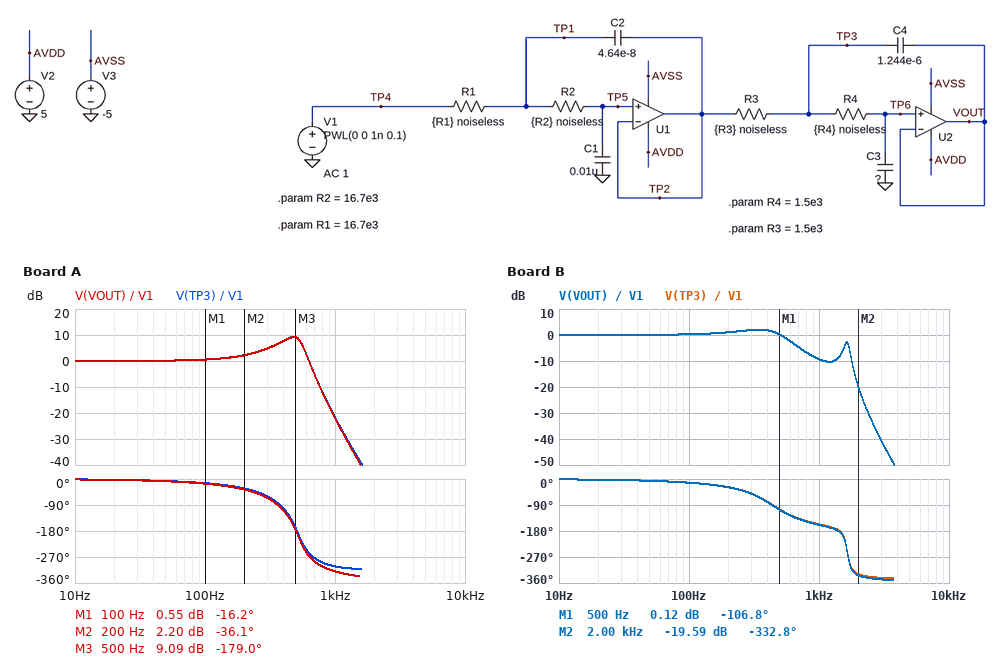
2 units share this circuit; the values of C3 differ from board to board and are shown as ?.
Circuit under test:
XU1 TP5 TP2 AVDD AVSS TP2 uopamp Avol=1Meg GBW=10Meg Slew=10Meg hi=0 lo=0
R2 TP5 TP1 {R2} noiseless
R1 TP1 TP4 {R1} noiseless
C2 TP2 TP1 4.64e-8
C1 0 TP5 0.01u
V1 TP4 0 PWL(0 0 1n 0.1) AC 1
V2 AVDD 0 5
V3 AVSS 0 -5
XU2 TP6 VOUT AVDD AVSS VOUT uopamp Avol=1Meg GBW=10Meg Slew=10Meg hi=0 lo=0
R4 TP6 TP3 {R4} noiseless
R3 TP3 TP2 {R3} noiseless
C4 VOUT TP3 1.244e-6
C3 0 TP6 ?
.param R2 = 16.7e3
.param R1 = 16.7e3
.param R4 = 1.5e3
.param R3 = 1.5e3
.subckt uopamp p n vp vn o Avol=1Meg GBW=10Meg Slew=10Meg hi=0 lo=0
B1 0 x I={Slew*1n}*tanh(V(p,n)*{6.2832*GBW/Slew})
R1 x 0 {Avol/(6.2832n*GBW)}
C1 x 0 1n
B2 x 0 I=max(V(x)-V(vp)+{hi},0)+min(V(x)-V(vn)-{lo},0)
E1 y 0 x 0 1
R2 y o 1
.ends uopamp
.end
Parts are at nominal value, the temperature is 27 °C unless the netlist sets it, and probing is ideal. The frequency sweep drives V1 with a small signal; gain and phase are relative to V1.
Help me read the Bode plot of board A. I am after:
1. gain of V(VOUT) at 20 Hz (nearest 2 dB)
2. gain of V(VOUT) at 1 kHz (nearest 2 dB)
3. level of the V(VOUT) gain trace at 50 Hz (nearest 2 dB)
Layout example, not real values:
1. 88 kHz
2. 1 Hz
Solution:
1. 0 dB
2. -22 dB
3. 0 dB
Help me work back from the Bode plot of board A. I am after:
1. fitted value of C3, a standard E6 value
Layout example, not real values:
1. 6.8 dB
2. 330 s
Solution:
1. 33 nF
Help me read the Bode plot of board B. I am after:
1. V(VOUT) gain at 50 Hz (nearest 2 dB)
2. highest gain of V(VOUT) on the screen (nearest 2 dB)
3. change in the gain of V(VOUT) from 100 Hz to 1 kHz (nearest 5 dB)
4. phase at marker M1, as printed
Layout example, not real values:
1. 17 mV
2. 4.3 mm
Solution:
1. 0 dB
2. 2 dB
3. -10 dB
4. -106.8 deg
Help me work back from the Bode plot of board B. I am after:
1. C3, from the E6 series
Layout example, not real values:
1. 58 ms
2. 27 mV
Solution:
1. 3.3 nF
